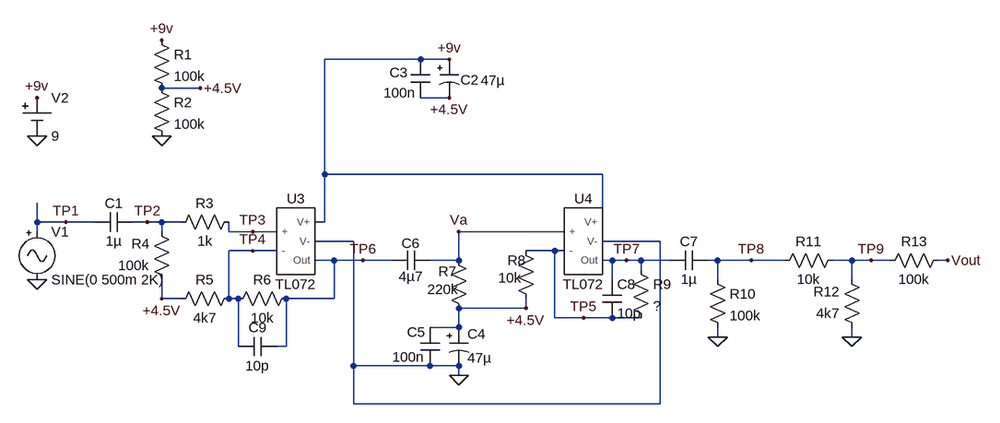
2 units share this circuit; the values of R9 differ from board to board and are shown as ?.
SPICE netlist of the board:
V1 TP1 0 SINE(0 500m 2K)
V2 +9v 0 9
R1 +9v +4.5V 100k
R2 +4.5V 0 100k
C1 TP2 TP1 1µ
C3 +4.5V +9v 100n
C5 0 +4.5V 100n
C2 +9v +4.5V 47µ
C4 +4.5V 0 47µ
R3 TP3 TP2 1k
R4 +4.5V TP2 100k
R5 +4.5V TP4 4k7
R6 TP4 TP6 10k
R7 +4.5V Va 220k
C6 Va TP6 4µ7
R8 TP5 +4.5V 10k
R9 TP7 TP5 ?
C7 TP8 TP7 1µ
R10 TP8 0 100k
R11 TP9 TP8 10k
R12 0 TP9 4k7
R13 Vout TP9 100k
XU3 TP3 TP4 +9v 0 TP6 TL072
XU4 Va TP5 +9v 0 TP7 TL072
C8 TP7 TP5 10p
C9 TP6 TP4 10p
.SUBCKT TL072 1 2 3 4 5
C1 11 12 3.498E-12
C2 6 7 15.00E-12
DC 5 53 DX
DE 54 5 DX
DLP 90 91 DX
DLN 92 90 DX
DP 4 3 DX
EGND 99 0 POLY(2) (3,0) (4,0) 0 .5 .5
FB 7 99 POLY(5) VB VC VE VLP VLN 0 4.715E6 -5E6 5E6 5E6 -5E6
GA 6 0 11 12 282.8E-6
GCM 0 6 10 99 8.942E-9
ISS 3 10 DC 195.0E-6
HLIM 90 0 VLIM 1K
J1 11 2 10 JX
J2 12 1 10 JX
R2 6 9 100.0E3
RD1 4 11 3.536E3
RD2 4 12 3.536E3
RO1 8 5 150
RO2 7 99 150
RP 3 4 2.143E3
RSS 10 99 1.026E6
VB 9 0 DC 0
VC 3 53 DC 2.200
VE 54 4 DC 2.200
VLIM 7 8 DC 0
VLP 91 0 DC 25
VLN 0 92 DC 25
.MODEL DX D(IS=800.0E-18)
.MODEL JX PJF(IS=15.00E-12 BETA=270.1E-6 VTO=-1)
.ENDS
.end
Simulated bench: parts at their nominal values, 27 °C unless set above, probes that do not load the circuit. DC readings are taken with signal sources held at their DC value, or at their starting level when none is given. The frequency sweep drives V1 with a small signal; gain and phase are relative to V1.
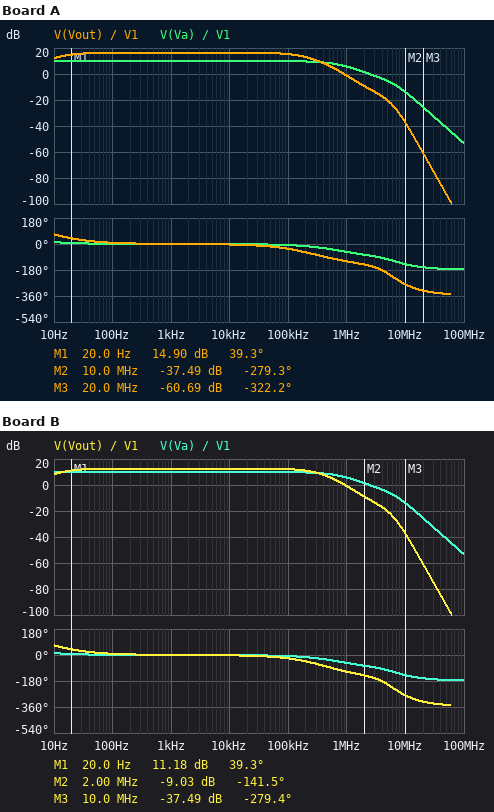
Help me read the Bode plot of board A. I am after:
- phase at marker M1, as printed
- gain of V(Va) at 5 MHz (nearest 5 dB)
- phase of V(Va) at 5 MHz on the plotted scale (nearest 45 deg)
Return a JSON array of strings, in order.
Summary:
["39.3 deg", "-5 dB", "-90 deg"]
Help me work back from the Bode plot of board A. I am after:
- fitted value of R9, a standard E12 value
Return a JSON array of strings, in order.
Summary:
["56 kΩ"]
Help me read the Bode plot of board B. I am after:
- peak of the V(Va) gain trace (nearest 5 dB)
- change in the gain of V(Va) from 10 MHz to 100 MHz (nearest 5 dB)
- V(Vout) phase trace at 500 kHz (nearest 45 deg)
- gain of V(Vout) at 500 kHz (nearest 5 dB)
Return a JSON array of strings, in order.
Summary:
["10 dB", "-40 dB", "-90 deg", "5 dB"]
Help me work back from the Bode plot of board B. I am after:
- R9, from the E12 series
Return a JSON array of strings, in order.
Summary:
["33 kΩ"]
